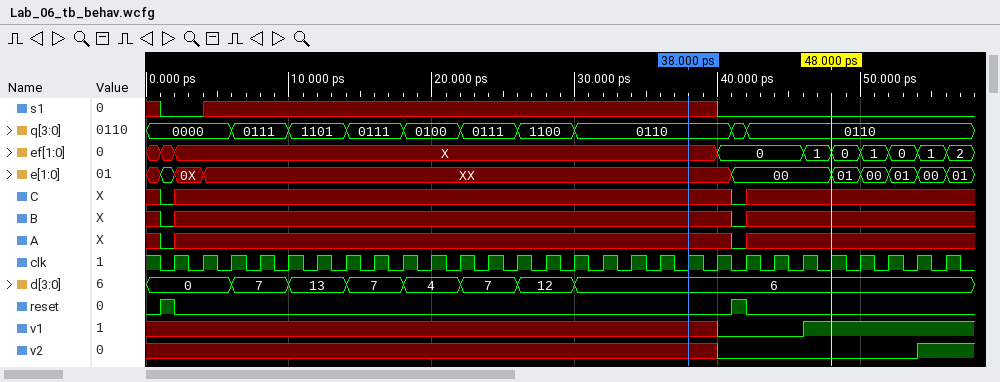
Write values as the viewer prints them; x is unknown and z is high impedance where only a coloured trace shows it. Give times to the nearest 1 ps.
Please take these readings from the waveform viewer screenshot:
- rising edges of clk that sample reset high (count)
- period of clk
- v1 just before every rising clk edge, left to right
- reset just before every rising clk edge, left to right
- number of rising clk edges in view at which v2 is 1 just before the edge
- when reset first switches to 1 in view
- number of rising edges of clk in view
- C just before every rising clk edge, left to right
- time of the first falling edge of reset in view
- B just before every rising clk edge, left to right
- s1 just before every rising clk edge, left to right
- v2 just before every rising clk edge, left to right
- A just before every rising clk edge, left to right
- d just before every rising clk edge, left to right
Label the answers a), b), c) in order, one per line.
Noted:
a) 2
b) 2 ps
c) x x x x x x x x x x x x x x x x x x x x 0 0 0 1 1 1 1 1
d) 1 0 0 0 0 0 0 0 0 0 0 0 0 0 0 0 0 0 0 0 1 0 0 0 0 0 0 0
e) 1
f) 1 ps
g) 28
h) 0 x x x x x x x x x x x x x x x x x x x 0 x x x x x x x
i) 2 ps
j) 0 x x x x x x x x x x x x x x x x x x x 0 x x x x x x x
k) 0 0 x x x x x x x x x x x x x x x x x x 0 0 0 0 0 0 0 0
l) x x x x x x x x x x x x x x x x x x x x 0 0 0 0 0 0 0 1
m) 0 x x x x x x x x x x x x x x x x x x x 0 x x x x x x x
n) 0, 0, 0, 7, 7, 13, 13, 7, 7, 4, 4, 7, 7, 12, 12, 6, 6, 6, 6, 6, 6, 6, 6, 6, 6, 6, 6, 6
